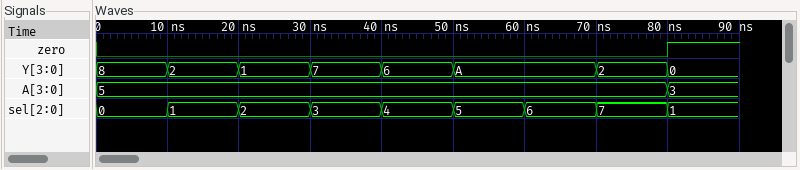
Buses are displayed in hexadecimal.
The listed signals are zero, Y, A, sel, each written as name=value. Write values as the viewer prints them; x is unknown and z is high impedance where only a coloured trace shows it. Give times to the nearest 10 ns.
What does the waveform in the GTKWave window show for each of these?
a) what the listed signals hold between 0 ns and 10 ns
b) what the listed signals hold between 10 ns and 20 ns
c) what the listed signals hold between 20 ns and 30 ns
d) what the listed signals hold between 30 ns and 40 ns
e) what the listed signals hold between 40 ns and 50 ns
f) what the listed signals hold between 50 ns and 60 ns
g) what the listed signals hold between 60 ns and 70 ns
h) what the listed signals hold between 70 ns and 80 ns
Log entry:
zero=0, Y=8, A=5, sel=0
zero=0, Y=2, A=5, sel=1
zero=0, Y=1, A=5, sel=2
zero=0, Y=7, A=5, sel=3
zero=0, Y=6, A=5, sel=4
zero=0, Y=A, A=5, sel=5
zero=0, Y=A, A=5, sel=6
zero=0, Y=2, A=5, sel=7
